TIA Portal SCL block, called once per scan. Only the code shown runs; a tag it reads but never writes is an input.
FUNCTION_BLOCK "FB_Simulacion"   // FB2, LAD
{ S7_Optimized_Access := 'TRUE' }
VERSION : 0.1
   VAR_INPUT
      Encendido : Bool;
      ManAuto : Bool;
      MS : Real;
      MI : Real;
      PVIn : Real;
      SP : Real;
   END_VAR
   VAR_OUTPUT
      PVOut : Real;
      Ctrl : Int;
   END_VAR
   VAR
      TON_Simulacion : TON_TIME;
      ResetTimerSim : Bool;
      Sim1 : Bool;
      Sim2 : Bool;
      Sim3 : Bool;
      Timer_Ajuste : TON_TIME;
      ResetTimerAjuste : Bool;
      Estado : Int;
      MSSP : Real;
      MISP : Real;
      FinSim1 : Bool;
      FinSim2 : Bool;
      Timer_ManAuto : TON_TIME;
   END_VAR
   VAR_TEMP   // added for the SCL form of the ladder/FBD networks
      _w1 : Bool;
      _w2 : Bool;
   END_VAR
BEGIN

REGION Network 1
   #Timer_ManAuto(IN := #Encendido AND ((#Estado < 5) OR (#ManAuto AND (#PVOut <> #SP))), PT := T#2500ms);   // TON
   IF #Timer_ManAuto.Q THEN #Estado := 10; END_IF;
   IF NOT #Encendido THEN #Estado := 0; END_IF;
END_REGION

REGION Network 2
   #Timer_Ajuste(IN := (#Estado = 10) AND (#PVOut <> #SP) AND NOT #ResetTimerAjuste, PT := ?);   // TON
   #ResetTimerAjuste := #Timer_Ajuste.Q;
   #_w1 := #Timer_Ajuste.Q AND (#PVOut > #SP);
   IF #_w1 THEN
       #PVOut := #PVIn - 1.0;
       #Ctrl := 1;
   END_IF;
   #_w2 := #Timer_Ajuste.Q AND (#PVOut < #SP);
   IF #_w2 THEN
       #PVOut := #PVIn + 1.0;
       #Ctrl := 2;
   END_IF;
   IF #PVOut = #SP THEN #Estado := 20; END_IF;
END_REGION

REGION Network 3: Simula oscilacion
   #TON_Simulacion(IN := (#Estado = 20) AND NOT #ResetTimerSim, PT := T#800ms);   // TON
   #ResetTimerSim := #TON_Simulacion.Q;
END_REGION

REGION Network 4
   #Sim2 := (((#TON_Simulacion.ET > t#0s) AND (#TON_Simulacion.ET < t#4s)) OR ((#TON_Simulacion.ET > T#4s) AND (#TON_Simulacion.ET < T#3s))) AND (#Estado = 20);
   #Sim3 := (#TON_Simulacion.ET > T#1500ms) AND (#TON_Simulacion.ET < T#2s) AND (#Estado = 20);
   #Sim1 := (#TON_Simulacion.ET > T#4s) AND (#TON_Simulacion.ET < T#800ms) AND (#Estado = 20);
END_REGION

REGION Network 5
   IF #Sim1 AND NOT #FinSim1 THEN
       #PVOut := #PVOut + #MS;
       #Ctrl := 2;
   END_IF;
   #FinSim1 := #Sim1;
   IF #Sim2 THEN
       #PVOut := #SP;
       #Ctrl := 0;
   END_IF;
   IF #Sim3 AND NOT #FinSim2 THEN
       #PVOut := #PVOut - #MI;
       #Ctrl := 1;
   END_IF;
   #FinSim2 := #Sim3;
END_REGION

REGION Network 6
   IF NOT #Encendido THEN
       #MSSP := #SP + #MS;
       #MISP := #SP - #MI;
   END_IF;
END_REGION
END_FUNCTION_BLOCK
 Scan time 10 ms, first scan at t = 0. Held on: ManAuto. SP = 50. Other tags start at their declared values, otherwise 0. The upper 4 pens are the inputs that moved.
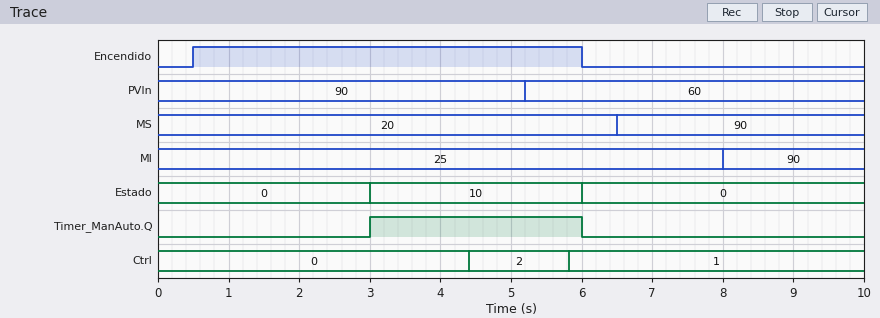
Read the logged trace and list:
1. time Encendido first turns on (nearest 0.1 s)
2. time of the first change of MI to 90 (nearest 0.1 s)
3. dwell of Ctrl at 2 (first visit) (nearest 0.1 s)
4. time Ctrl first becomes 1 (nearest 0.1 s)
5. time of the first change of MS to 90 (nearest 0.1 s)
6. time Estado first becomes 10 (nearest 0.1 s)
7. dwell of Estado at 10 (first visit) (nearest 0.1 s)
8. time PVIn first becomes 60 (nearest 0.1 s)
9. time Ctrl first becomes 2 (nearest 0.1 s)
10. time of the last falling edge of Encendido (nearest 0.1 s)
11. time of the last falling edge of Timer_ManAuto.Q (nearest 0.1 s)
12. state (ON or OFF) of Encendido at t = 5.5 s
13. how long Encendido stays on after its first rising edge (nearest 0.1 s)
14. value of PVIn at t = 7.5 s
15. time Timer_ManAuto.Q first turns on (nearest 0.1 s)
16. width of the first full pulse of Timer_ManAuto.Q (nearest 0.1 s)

0.5 s
8.0 s
1.4 s
5.8 s
6.5 s
3.0 s
3.0 s
5.2 s
4.4 s
6.0 s
6.0 s
ON
5.5 s
60
3.0 s
3.0 s
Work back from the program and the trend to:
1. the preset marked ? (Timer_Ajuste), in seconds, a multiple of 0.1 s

1.4 s
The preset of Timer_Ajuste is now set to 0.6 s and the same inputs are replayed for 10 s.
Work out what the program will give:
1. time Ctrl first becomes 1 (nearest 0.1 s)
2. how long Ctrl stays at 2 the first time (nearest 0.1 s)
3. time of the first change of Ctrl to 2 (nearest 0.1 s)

4.2 s
0.6 s
3.6 s
